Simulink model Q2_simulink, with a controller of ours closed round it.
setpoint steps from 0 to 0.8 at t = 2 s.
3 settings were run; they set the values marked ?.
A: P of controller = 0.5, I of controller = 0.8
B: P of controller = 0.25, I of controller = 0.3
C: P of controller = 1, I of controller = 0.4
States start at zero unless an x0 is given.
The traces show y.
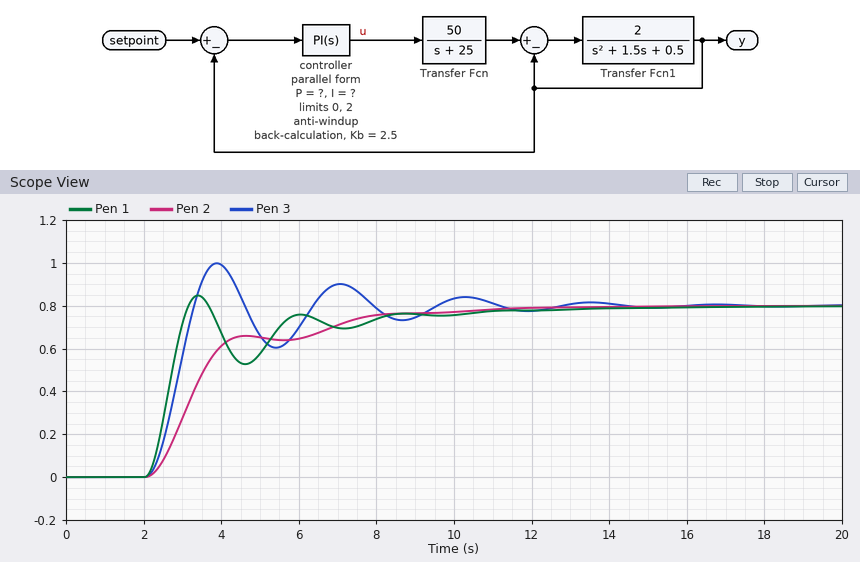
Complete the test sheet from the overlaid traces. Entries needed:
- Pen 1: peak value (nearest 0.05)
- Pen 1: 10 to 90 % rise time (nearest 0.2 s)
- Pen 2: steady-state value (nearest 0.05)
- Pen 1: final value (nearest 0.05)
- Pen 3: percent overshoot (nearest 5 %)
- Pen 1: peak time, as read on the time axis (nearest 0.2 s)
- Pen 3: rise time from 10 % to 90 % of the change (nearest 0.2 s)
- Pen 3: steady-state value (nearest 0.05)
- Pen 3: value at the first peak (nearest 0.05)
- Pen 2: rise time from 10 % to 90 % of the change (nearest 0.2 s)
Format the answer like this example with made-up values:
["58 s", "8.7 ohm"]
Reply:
["0.85", "0.8 s", "0.80", "0.80", "25 %", "3.4 s", "0.8 s", "0.80", "1.00", "4.6 s"]
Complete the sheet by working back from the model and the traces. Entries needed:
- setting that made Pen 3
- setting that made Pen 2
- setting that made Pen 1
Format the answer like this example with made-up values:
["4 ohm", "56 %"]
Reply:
["A", "B", "C"]
